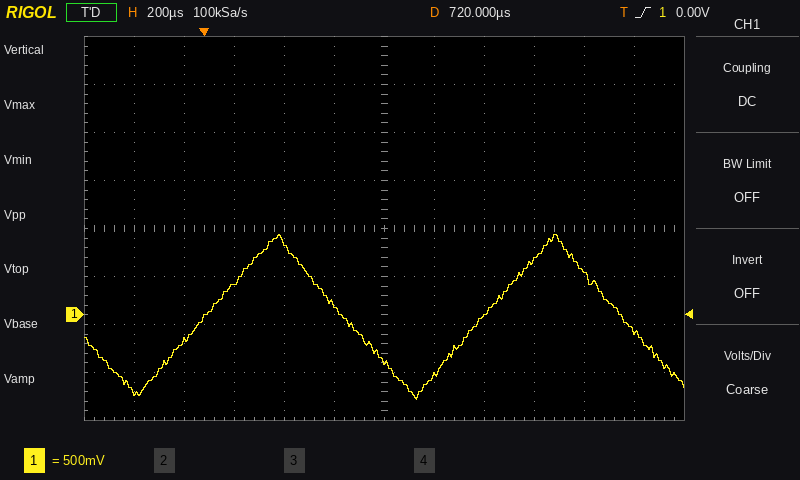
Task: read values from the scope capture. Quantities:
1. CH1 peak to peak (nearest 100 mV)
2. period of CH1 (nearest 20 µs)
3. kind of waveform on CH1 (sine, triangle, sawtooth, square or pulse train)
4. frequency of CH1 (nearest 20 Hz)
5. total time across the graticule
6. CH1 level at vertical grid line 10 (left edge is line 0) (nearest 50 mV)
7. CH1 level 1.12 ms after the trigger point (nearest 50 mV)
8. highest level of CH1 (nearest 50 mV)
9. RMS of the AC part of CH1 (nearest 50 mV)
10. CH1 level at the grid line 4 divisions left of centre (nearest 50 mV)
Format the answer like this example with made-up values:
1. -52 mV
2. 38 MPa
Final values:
1. 1.70 V
2. 1.12 ms
3. triangle
4. 900 Hz
5. 2.4 ms
6. 450 mV
7. 0 mV
8. 850 mV
9. 500 mV
10. -300 mV
